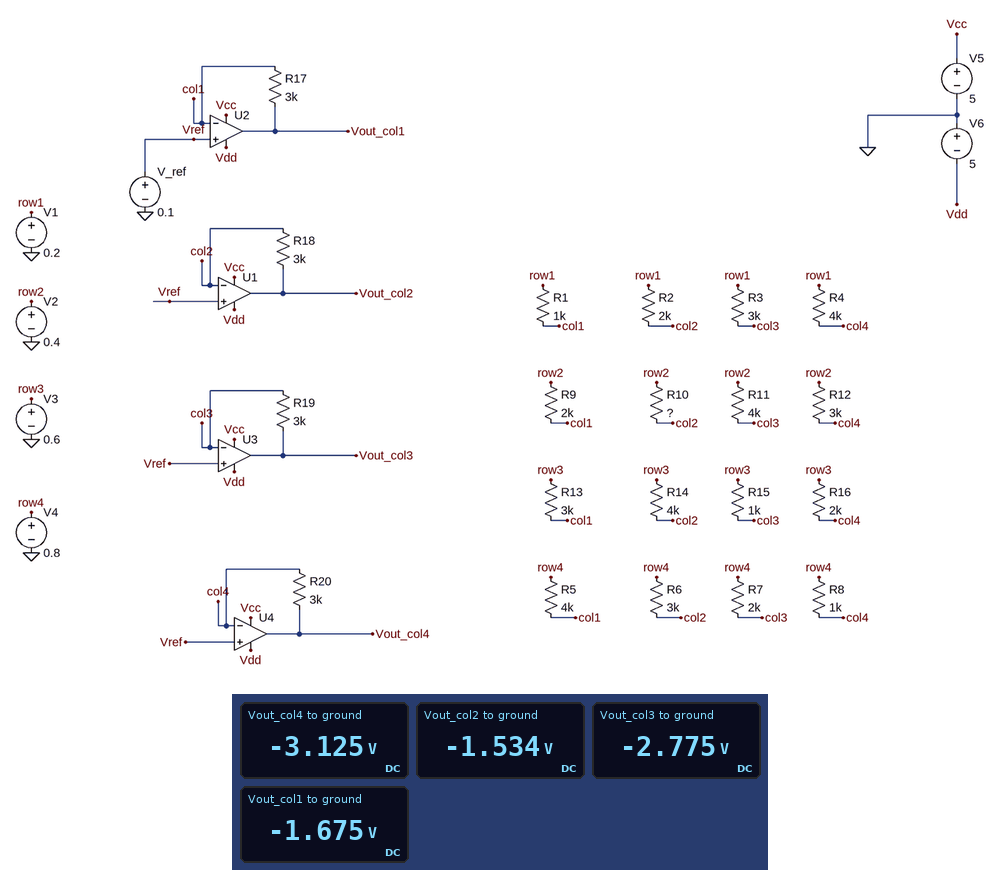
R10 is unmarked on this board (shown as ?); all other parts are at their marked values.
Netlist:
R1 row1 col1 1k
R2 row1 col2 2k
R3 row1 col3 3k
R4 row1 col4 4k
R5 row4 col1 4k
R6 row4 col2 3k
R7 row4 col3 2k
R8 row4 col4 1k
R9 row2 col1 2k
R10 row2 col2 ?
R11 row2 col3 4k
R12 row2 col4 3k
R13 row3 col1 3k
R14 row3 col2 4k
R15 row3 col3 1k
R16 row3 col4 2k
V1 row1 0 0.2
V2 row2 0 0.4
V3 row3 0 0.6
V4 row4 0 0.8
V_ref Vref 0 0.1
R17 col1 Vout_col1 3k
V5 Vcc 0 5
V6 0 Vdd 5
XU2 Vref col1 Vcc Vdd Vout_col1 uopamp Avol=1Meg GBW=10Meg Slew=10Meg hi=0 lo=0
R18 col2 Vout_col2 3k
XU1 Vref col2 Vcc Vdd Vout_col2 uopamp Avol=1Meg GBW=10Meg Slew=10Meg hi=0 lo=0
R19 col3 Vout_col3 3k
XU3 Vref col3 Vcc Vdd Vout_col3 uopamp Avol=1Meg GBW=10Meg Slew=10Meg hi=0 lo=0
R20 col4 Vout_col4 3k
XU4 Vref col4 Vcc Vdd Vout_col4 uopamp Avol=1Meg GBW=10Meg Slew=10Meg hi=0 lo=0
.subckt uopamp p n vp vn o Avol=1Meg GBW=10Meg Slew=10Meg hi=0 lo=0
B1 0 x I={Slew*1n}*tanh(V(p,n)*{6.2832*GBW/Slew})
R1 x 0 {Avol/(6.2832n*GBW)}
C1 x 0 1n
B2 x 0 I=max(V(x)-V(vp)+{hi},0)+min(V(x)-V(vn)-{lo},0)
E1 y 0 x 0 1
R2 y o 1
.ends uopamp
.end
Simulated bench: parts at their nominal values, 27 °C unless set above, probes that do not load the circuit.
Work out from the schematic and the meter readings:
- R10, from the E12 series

2.2 kΩ
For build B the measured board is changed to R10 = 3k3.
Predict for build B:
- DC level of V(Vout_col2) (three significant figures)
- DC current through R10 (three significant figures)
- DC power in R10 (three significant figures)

-1.40 V
90.9 µA
27.3 µW
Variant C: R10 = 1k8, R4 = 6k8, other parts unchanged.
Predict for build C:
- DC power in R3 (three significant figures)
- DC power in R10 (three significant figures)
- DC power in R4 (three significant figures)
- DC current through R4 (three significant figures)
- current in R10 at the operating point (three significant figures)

3.33 µW
50.0 µW
1.47 µW
14.7 µA
167 µA
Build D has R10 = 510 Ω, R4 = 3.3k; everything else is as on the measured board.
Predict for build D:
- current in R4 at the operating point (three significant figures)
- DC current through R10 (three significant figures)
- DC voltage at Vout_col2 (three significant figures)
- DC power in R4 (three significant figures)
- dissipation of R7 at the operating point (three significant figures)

30.3 µA
588 µA
-2.89 V
3.03 µW
245 µW
